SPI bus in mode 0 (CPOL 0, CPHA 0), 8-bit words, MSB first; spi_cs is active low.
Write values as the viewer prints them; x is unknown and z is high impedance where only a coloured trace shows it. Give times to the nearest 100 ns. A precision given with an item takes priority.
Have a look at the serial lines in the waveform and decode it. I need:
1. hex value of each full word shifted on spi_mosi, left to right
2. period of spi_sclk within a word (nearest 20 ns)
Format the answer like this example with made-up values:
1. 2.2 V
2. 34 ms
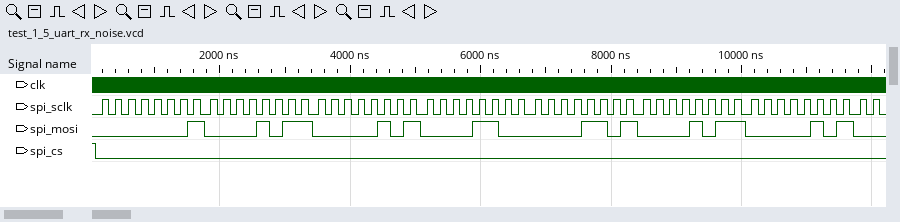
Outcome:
1. 01, 0B, 05, 0C, 0D, 0B, 05
2. 200 ns
